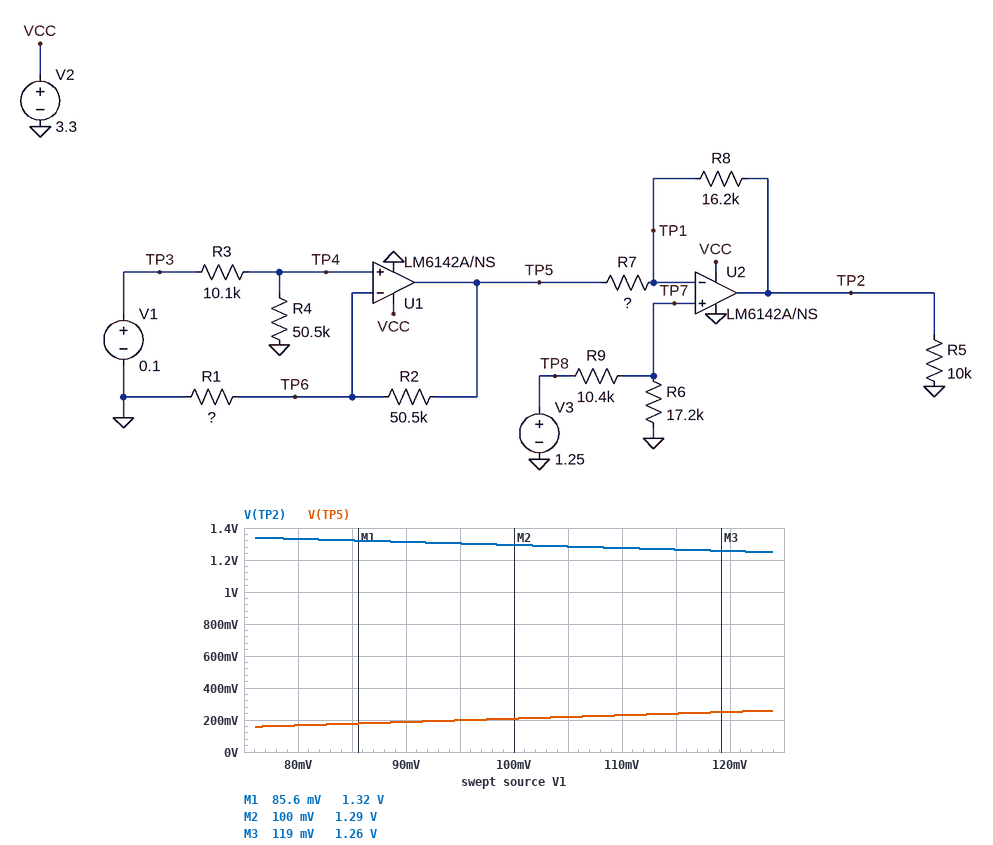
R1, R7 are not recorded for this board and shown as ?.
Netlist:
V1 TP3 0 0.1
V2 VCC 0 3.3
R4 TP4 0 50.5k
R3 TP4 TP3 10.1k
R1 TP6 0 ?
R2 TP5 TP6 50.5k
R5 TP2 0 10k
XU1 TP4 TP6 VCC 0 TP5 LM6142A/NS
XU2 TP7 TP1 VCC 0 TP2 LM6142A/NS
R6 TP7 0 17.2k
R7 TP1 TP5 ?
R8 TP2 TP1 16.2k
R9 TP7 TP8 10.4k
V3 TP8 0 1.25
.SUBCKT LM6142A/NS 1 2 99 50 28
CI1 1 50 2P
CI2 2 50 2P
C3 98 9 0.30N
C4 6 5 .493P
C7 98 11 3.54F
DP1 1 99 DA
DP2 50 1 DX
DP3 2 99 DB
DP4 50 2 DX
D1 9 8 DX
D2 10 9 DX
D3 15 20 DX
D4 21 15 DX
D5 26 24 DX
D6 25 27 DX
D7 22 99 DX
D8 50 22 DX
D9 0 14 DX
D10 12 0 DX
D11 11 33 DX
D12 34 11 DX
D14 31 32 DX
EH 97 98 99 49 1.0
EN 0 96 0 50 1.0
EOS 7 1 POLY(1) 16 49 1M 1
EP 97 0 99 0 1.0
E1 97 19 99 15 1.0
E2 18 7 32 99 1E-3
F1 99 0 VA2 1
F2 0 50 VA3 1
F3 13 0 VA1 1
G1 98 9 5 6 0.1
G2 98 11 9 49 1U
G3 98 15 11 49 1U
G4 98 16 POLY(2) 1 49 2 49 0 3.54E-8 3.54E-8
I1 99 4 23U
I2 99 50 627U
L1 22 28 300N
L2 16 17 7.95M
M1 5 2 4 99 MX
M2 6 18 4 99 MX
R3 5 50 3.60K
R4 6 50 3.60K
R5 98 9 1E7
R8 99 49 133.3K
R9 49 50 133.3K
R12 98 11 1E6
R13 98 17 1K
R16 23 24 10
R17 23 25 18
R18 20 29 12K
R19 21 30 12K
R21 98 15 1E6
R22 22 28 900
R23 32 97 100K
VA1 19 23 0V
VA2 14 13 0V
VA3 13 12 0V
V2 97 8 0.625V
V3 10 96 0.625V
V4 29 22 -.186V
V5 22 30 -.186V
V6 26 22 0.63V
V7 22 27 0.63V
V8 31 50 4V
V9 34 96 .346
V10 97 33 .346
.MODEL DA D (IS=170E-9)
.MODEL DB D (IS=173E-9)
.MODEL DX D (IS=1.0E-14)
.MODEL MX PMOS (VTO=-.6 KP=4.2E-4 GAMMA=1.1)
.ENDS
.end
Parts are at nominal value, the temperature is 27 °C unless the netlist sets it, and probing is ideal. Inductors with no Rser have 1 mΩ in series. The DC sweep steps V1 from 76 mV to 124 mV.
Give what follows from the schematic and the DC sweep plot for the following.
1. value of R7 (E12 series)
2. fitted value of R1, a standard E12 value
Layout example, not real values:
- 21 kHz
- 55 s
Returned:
- 18 kΩ
- 33 kΩ
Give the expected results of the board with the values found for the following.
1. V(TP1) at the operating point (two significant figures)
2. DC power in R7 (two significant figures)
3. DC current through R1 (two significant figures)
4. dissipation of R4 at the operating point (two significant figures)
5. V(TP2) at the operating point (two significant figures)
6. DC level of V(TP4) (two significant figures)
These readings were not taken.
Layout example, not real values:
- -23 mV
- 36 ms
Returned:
- 780 mV
- 18 µW
- 2.6 µA
- 140 nW
- 1.3 V
- 85 mV
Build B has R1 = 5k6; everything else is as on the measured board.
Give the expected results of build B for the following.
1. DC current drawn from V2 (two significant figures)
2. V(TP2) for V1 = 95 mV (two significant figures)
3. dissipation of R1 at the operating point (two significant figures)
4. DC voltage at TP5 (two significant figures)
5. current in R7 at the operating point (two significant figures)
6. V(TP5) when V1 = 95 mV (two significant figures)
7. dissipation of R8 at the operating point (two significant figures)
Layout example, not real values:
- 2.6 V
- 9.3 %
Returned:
- 1.4 mA
- 750 mV
- 1.3 µW
- 850 mV
- 3.9 µA
- 810 mV
- 270 nW
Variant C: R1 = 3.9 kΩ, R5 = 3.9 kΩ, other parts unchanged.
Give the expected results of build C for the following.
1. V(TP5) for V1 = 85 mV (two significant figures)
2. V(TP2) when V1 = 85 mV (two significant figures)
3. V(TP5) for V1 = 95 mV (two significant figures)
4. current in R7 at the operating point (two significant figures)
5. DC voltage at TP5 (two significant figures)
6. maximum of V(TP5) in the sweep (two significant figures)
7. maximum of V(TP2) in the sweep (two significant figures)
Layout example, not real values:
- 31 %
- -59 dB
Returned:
- 1.0 V
- 570 mV
- 1.1 V
- 23 µA
- 1.2 V
- 1.5 V
- 660 mV
